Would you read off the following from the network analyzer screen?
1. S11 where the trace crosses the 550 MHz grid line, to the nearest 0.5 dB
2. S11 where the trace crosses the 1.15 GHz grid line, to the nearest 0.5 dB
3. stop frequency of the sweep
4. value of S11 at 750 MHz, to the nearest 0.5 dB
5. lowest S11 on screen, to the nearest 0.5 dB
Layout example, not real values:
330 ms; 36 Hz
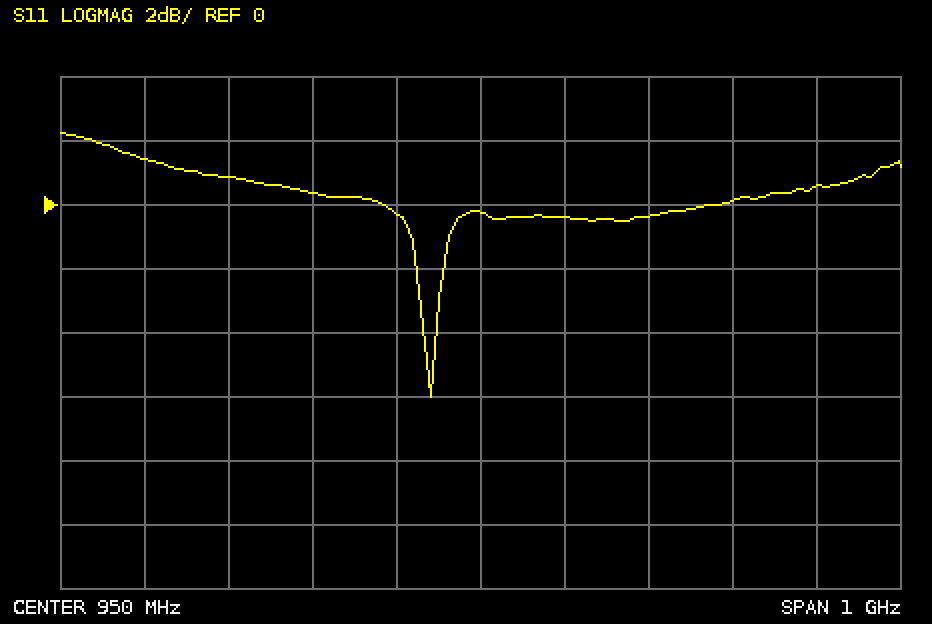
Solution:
1.5 dB; -0.5 dB; 1.45 GHz; 0.5 dB; -6.0 dB
